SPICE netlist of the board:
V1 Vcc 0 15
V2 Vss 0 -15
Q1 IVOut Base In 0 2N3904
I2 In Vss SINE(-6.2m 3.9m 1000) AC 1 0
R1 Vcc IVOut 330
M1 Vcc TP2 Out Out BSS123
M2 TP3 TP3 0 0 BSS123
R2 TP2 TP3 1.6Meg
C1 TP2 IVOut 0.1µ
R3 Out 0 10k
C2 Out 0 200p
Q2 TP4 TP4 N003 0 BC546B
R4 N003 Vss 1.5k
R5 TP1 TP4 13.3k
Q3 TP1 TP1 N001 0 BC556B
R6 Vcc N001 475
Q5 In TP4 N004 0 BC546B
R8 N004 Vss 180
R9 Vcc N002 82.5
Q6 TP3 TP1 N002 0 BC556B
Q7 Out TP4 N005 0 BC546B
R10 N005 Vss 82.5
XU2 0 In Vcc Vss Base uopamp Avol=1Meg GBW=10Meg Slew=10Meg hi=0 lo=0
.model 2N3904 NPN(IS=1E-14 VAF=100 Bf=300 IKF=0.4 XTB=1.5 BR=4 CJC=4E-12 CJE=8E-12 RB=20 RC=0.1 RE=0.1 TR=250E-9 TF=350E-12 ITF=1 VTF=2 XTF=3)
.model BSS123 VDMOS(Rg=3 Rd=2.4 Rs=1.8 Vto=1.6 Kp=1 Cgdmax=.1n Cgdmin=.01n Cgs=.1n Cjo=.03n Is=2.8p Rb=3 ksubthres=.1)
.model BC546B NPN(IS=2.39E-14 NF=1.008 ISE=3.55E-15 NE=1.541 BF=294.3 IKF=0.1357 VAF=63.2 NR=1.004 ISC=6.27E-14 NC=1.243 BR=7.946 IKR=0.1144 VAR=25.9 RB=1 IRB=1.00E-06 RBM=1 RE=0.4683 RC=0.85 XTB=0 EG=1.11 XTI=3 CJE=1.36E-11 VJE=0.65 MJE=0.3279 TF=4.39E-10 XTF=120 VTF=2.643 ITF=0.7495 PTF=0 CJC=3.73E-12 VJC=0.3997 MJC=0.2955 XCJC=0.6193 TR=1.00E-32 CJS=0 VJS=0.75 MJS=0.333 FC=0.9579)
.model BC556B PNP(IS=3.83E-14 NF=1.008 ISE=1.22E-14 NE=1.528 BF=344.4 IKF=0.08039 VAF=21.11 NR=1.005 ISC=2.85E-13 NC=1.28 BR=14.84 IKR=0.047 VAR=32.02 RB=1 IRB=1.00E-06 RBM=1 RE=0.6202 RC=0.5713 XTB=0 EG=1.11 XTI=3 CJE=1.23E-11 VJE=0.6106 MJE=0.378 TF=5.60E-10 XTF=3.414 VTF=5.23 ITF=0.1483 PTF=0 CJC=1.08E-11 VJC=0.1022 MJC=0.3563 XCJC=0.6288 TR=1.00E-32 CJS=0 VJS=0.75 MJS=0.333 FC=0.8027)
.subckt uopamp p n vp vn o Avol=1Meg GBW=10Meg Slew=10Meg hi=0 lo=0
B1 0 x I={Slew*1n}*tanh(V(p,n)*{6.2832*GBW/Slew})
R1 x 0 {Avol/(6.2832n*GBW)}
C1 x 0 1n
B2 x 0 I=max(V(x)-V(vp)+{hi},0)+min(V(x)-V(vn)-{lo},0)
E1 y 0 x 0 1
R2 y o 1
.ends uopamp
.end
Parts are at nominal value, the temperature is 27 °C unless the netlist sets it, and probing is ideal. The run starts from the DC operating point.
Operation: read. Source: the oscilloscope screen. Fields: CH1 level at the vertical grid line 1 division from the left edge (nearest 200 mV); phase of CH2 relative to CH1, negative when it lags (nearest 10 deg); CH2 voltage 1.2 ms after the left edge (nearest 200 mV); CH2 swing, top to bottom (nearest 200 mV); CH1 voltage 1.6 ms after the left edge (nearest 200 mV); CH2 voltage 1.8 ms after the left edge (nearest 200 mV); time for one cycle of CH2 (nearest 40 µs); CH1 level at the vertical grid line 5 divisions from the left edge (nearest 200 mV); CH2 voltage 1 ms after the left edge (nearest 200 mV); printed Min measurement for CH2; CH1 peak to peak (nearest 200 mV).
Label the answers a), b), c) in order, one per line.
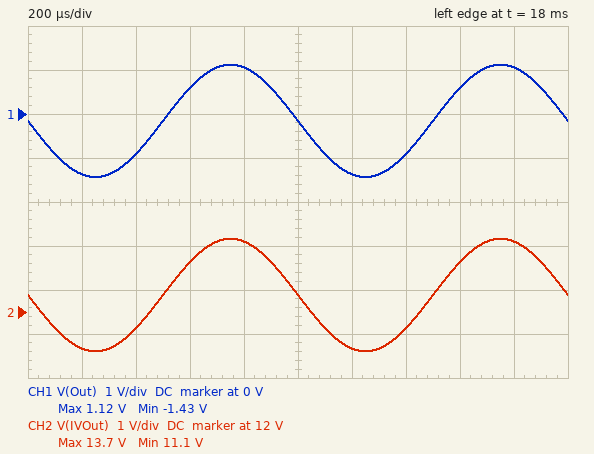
a) -1.4 V
b) 0 deg
c) 11.2 V
d) 2.6 V
e) 600 mV
f) 13.6 V
g) 1.00 ms
h) -200 mV
i) 12.4 V
j) 11.1 V
k) 2.6 V
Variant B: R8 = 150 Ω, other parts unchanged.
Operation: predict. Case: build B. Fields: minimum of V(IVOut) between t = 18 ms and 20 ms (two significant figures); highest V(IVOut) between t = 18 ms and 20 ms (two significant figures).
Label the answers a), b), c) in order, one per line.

a) 10 V
b) 13 V
